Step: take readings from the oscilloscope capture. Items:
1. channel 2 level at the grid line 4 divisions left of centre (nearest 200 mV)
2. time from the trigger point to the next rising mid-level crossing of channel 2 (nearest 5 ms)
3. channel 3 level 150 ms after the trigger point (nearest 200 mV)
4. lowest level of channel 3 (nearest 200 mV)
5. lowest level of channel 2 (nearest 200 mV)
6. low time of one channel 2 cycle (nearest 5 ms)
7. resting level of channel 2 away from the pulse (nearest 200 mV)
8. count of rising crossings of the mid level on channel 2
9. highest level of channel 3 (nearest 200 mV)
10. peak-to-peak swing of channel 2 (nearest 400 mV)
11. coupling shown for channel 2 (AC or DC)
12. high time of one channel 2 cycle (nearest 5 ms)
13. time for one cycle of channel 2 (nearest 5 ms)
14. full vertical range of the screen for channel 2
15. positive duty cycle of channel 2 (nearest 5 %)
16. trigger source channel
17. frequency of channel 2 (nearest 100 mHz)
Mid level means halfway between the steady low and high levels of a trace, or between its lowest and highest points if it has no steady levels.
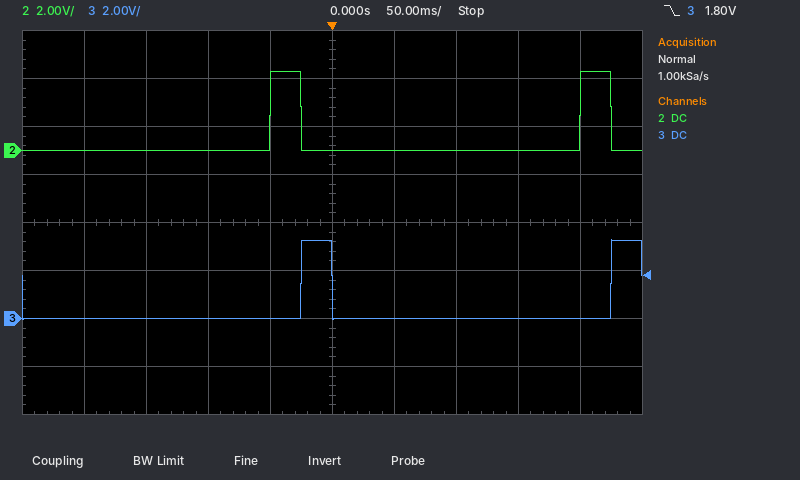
0.0 V
200 ms
0.0 V
0.0 V
0.0 V
225 ms
0.0 V
2
3.2 V
3.2 V
DC
25 ms
250 ms
16 V
10 %
channel 3
4.0 Hz
